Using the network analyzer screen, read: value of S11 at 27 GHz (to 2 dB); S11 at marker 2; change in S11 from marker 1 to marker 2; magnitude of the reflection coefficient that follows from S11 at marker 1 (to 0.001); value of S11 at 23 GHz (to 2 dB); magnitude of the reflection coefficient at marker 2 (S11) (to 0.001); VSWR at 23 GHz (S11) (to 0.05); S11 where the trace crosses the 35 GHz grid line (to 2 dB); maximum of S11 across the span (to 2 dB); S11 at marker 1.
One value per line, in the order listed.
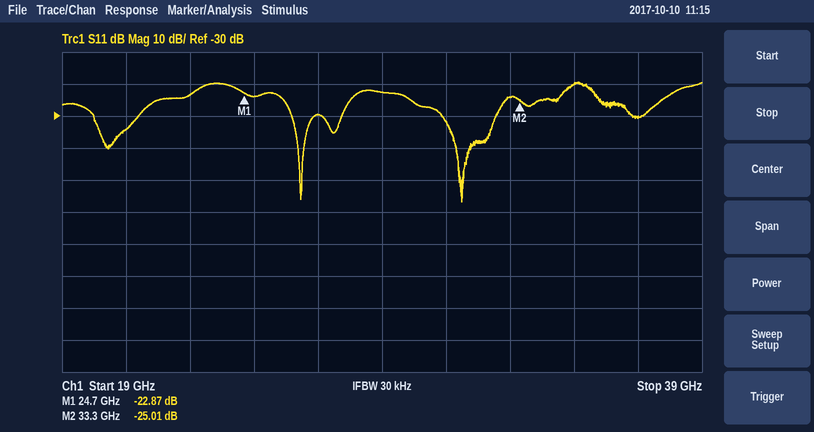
-30 dB
-25.01 dB
-2.14 dB
0.072
-24 dB
0.056
1.15
-20 dB
-20 dB
-22.87 dB
